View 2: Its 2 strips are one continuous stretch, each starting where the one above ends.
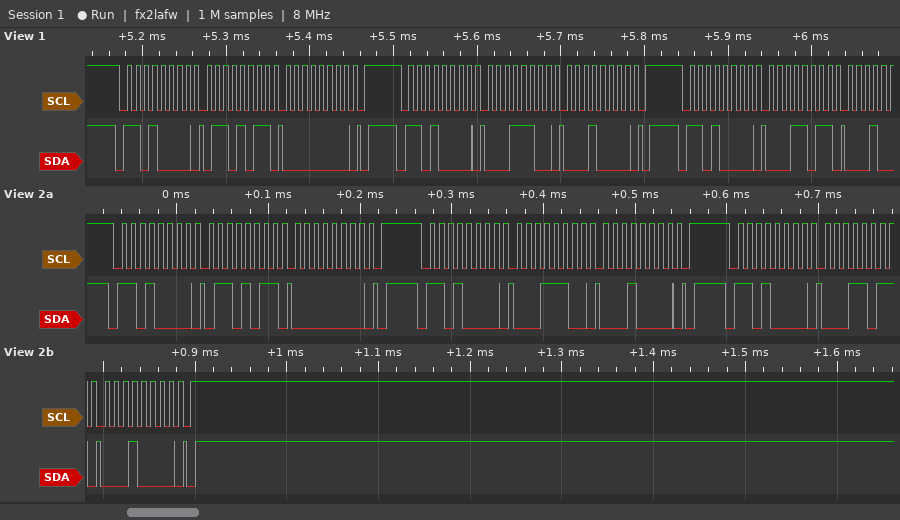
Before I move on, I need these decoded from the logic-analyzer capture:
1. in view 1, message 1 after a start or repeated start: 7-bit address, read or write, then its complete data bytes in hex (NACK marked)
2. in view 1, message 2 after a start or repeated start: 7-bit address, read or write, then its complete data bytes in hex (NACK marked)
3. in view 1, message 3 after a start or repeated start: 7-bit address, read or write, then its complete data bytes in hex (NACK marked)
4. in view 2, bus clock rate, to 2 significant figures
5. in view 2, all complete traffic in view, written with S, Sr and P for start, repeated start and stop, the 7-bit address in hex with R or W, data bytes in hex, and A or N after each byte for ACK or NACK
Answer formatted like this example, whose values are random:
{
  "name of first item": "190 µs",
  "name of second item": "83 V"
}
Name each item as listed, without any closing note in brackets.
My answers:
{
  "in view 1, message 1 after a start or repeated start: 7-bit address, read or write, then its complete data bytes in hex": "0x68 write: 6B 00",
  "in view 1, message 2 after a start or repeated start: 7-bit address, read or write, then its complete data bytes in hex": "0x68 write: 1C 10",
  "in view 1, message 3 after a start or repeated start: 7-bit address, read or write, then its complete data bytes in hex": "0x68 write: 1B",
  "in view 2, bus clock rate, to 2 significant figures": "100 kHz",
  "in view 2, all complete traffic in view, written with S, Sr and P for start, repeated start and stop, the 7-bit address in hex with R or W, data bytes in hex, and A or N after each byte for ACK or NACK": "S 68W A 6B A 00 A P S 68W A 1C A 10 A P S 68W A 1B A 10 A P"
}
